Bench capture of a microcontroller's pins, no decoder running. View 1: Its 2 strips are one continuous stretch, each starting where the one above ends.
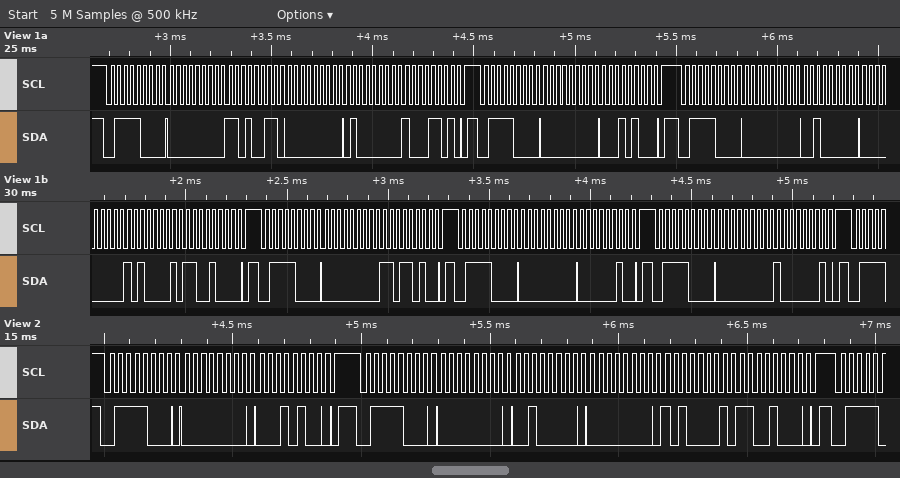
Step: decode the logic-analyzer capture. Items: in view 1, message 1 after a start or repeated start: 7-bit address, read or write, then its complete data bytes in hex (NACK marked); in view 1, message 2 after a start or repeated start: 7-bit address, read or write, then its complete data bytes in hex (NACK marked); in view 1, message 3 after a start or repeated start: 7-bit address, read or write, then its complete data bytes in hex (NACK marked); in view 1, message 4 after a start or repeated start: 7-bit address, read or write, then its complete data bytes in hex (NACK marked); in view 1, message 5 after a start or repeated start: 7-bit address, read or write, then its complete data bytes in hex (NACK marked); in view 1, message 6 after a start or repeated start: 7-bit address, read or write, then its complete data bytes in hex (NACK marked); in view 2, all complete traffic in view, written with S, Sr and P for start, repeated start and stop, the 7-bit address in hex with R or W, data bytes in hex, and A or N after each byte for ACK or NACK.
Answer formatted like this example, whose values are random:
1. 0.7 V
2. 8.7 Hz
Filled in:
1. 0x3C write: 00 D3 00 40 8D
2. 0x3C write: 00 14
3. 0x3C write: 00 20 00 A1 C8
4. 0x3C write: 00 DA
5. 0x3C write: 00 02
6. 0x3C write: 00 81
7. S 3CW A 00 A 14 A P S 3CW A 00 A 20 A 00 A A1 A C8 A P
